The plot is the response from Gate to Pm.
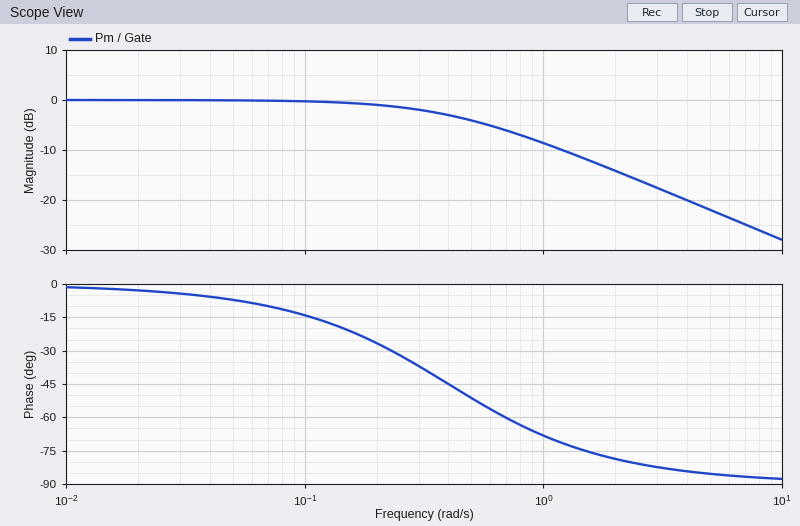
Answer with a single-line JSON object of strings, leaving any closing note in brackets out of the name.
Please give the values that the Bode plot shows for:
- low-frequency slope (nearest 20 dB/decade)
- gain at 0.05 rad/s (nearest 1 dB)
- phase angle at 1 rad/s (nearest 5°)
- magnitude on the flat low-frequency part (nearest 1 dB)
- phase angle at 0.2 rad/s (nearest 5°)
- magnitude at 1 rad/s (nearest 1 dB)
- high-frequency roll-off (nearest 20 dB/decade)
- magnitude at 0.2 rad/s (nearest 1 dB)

{"low-frequency slope": "0 dB/decade", "gain at 0.05 rad/s": "0 dB", "phase angle at 1 rad/s": "-70°", "magnitude on the flat low-frequency part": "0 dB", "phase angle at 0.2 rad/s": "-25°", "magnitude at 1 rad/s": "-9 dB", "high-frequency roll-off": "-20 dB/decade", "magnitude at 0.2 rad/s": "-1 dB"}
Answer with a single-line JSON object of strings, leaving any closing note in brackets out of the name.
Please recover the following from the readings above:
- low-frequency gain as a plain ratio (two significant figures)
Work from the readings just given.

{"low-frequency gain as a plain ratio": "1.0"}
